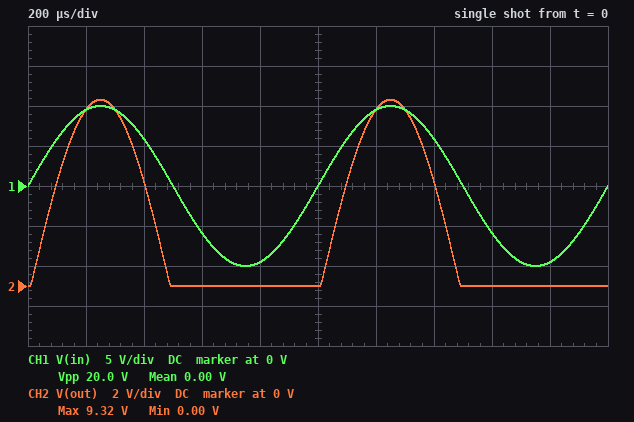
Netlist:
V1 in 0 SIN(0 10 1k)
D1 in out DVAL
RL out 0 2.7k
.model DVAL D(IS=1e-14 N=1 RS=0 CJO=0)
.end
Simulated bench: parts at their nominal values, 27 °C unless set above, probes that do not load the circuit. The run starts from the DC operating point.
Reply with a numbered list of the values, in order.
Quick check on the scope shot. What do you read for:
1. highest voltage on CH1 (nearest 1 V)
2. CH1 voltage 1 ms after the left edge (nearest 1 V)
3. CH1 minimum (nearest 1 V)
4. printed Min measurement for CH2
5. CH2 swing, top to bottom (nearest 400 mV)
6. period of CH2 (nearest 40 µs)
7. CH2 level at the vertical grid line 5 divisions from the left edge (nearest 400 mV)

1. 10 V
2. 0 V
3. -10 V
4. 0.00 V
5. 9.2 V
6. 1.00 ms
7. 0 V
